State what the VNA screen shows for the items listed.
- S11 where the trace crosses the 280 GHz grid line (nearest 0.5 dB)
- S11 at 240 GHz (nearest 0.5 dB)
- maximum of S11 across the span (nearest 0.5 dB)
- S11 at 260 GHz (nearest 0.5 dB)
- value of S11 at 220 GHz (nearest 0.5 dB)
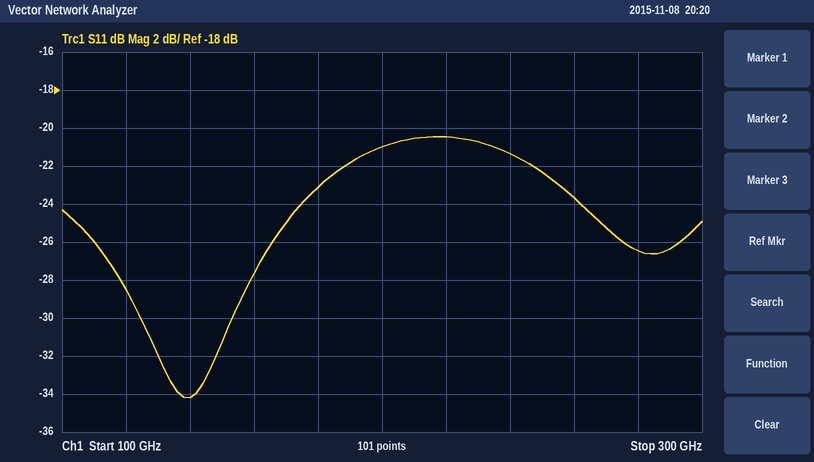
-26.5 dB
-21.5 dB
-20.5 dB
-23.5 dB
-20.5 dB
